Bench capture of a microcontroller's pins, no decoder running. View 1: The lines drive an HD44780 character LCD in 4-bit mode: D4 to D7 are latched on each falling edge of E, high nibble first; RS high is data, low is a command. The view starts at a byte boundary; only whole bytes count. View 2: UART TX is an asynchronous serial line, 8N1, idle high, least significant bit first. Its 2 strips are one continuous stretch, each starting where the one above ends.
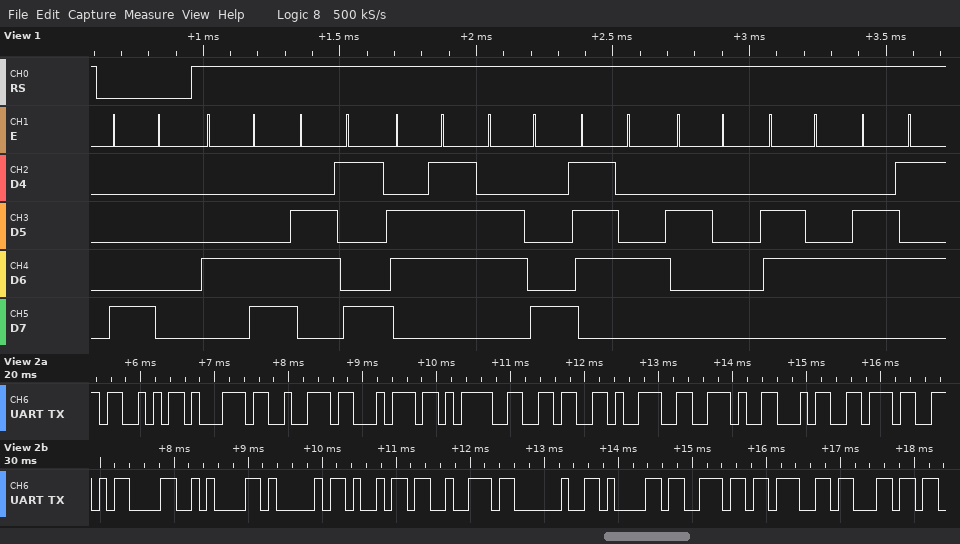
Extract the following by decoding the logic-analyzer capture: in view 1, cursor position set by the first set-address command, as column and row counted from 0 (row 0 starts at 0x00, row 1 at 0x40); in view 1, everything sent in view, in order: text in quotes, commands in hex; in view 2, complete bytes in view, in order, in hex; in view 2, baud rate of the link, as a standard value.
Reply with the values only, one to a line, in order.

column 0, row 0
0x80 "Light de"
0x53 0x71 0x72 0x74 0x3D 0x36 0x39 0x2E 0x34 0x37 0x0D 0x0A 0x41 0x69 0x72 0x20 0x61 0x6E 0x67 0x6C
9600 baud
